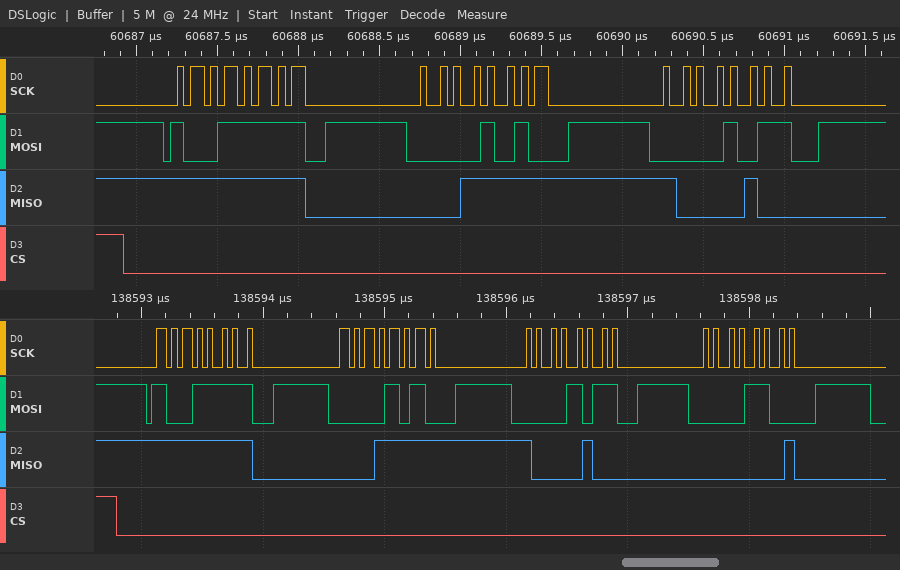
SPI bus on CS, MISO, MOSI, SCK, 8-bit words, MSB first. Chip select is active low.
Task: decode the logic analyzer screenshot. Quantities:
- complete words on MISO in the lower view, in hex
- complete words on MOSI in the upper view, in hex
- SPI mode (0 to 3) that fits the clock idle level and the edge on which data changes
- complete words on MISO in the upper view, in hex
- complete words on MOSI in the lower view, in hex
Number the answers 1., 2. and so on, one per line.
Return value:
1. FF, 1F, 84, 01
2. 9F, 0A, 0B
3. 0
4. FF, 1F, 84
5. 9F, 0A, 0B, 0C
